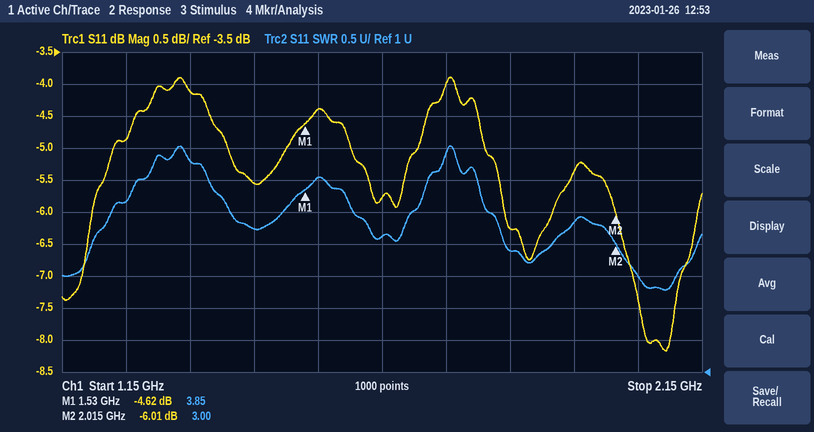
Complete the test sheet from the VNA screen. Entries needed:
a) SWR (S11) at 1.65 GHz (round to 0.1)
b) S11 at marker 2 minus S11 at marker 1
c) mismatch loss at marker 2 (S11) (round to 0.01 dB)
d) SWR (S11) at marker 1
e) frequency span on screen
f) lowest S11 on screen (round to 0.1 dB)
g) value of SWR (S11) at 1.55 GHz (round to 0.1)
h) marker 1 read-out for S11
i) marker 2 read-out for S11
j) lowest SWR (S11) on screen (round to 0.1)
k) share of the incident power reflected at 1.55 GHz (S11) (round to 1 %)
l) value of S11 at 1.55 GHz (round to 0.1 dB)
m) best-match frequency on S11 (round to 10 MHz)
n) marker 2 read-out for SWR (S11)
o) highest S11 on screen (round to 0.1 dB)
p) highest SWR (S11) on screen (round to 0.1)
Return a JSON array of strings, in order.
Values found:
["3.1", "-1.39 dB", "1.25 dB", "3.85", "1 GHz", "-8.2 dB", "4.0", "-4.62 dB", "-6.01 dB", "2.3", "36 %", "-4.4 dB", "2.09 GHz", "3.00", "-3.9 dB", "4.5"]
